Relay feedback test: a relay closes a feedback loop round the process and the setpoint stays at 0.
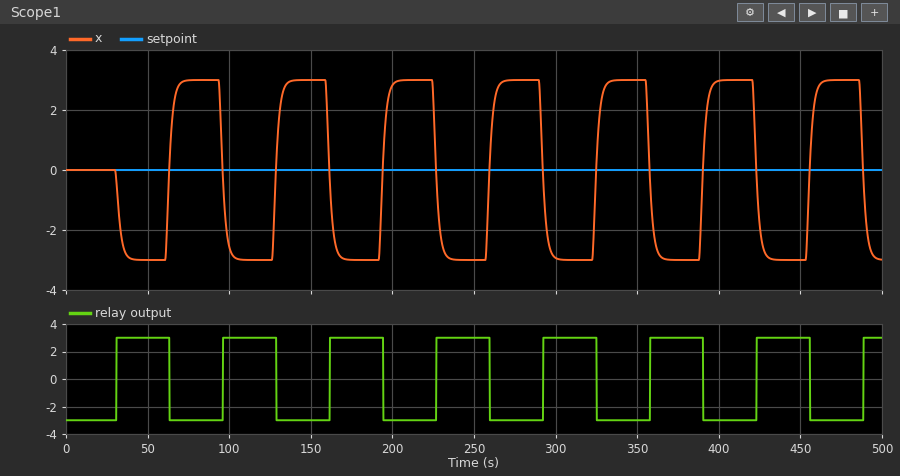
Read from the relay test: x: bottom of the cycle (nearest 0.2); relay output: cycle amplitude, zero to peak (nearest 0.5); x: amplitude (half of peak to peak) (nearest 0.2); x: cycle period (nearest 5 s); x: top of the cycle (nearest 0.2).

-3.0
3.0
3.0
65 s
3.0
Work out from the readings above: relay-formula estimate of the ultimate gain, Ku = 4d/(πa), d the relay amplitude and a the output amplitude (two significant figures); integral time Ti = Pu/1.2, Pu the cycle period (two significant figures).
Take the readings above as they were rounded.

1.3
54 s
